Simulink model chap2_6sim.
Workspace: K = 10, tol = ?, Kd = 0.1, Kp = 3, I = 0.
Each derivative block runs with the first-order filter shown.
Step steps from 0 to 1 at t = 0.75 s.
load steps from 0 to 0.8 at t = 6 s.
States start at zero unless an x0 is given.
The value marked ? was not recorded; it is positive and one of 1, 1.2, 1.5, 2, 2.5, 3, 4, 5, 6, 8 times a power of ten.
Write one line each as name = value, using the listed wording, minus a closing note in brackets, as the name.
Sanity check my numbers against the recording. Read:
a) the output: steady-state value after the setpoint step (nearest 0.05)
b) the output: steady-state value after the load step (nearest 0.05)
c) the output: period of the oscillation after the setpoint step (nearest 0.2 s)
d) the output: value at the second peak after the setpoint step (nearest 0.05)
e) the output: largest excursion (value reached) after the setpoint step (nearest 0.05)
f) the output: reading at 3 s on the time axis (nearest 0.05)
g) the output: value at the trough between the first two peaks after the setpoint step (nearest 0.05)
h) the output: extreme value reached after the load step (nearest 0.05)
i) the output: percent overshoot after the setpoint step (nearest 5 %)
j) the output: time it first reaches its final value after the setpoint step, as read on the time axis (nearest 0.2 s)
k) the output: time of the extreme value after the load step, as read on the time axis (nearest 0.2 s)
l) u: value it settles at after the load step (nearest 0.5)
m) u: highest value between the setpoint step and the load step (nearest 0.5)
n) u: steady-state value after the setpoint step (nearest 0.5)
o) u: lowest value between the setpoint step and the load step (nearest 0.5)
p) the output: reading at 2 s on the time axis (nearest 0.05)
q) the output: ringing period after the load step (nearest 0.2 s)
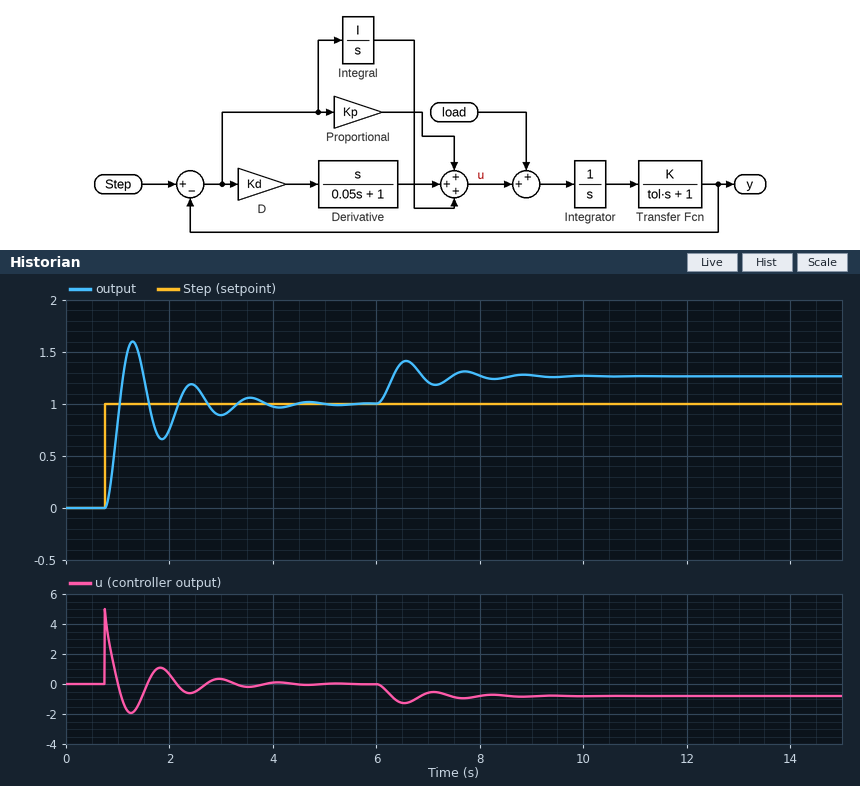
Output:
the output: steady-state value after the setpoint step = 1.00
the output: steady-state value after the load step = 1.25
the output: period of the oscillation after the setpoint step = 1.2 s
the output: value at the second peak after the setpoint step = 1.20
the output: largest excursion (value reached) after the setpoint step = 1.60
the output: reading at 3 s on the time axis = 0.90
the output: value at the trough between the first two peaks after the setpoint step = 0.65
the output: extreme value reached after the load step = 1.40
the output: percent overshoot after the setpoint step = 60 %
the output: time it first reaches its final value after the setpoint step, as read on the time axis = 1.0 s
the output: time of the extreme value after the load step, as read on the time axis = 6.6 s
u: value it settles at after the load step = -1.0
u: highest value between the setpoint step and the load step = 5.0
u: steady-state value after the setpoint step = 0.0
u: lowest value between the setpoint step and the load step = -2.0
the output: reading at 2 s on the time axis = 0.75
the output: ringing period after the load step = 1.2 s
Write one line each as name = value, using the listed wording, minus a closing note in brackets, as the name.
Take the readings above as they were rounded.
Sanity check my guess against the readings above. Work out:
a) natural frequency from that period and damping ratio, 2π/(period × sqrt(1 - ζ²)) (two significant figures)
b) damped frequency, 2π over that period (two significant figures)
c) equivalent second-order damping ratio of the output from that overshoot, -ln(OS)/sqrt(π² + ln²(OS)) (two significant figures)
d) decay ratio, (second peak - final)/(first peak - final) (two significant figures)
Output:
natural frequency from that period and damping ratio, 2π/(period × sqrt(1 - ζ²)) = 5.3 rad/s
damped frequency, 2π over that period = 5.2 rad/s
equivalent second-order damping ratio of the output from that overshoot, -ln(OS)/sqrt(π² + ln²(OS)) = 0.16
decay ratio, (second peak - final)/(first peak - final) = 0.33
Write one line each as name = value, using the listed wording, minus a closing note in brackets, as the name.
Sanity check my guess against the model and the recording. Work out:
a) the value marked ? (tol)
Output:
the value marked ? = 1
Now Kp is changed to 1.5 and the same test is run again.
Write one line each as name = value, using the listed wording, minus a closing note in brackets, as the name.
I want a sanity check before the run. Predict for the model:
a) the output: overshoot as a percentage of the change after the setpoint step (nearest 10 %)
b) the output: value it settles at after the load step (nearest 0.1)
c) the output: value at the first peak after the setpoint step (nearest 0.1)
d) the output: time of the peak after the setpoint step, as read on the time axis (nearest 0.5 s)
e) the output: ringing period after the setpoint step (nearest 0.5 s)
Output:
the output: overshoot as a percentage of the change after the setpoint step = 50 %
the output: value it settles at after the load step = 1.5
the output: value at the first peak after the setpoint step = 1.5
the output: time of the peak after the setpoint step, as read on the time axis = 1.5 s
the output: ringing period after the setpoint step = 1.5 s
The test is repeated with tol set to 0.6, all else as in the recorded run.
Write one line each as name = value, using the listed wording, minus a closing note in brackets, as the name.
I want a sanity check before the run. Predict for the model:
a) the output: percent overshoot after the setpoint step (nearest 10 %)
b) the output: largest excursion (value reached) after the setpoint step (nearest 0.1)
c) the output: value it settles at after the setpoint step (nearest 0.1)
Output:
the output: percent overshoot after the setpoint step = 50 %
the output: largest excursion (value reached) after the setpoint step = 1.5
the output: value it settles at after the setpoint step = 1.0
